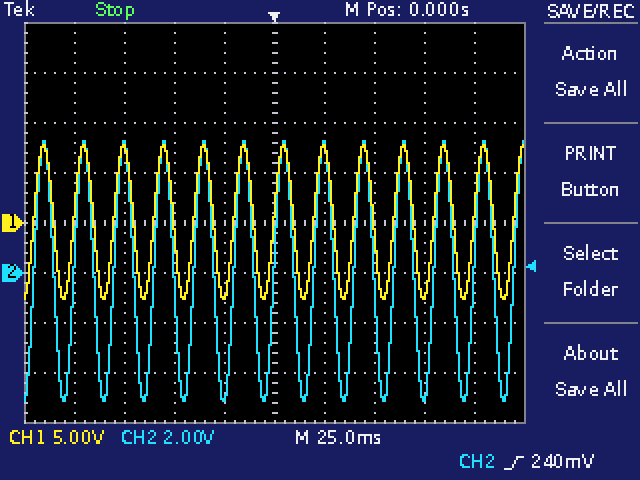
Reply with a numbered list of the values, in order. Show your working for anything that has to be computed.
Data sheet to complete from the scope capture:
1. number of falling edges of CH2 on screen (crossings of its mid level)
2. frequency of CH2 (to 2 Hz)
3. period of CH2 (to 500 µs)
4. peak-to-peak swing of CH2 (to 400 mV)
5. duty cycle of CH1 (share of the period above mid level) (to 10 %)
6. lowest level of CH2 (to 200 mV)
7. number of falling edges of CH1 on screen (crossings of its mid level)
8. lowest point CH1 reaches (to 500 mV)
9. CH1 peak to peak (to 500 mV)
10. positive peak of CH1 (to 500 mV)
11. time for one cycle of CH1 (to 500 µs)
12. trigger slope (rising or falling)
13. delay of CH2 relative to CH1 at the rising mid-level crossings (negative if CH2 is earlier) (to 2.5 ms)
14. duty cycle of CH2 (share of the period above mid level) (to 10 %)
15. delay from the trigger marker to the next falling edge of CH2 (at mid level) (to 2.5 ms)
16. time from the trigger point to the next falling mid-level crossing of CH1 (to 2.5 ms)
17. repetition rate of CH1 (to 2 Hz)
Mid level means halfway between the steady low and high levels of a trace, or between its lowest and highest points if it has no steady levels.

1. 12
2. 1 / 20.0 ms ≈ 50 Hz
3. 20.0 ms
4. 10.4 V
5. 50 %
6. -5.2 V
7. 12
8. -7.5 V
9. 8.0 V − (-7.5 V) = 15.5 V
10. 8.0 V
11. 20.0 ms
12. rising
13. 0.0 ms
14. 50 %
15. 10.0 ms
16. 10.0 ms
17. 1 / 20.0 ms ≈ 50 Hz
